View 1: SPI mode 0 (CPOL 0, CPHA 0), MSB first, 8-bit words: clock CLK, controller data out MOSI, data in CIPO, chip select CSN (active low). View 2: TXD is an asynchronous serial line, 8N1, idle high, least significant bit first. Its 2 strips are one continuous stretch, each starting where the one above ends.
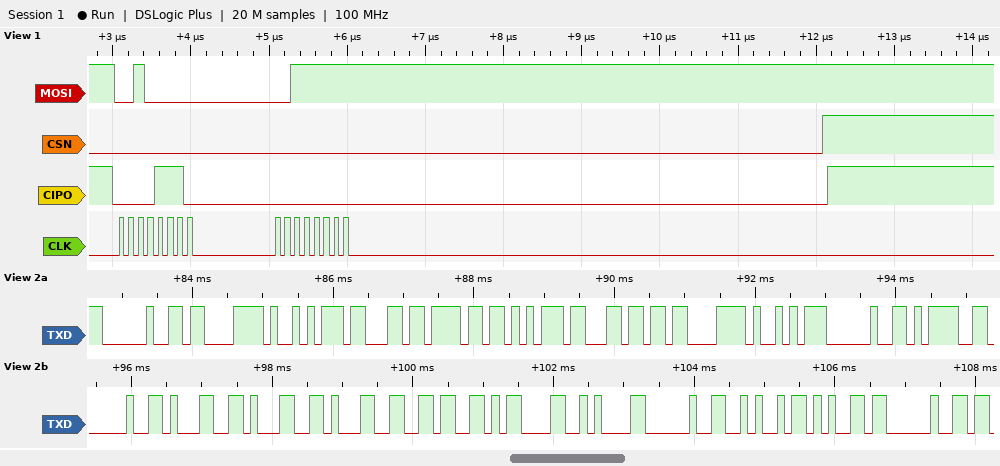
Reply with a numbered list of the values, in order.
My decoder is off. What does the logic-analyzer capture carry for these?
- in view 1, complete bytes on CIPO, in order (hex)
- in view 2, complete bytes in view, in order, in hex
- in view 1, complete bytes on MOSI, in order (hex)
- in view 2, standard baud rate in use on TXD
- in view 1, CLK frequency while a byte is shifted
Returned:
1. 0E 00
2. 0x20 0xC3 0xA9 0x63 0x6F 0x75 0x6C 0xC3 0xA9 0x20 0x3D 0x20 0x31 0x31 0x31 0x36 0x0D 0x0A 0x20 0x4A 0x65 0x20
3. 20 3F
4. 9600 baud
5. 8 MHz
